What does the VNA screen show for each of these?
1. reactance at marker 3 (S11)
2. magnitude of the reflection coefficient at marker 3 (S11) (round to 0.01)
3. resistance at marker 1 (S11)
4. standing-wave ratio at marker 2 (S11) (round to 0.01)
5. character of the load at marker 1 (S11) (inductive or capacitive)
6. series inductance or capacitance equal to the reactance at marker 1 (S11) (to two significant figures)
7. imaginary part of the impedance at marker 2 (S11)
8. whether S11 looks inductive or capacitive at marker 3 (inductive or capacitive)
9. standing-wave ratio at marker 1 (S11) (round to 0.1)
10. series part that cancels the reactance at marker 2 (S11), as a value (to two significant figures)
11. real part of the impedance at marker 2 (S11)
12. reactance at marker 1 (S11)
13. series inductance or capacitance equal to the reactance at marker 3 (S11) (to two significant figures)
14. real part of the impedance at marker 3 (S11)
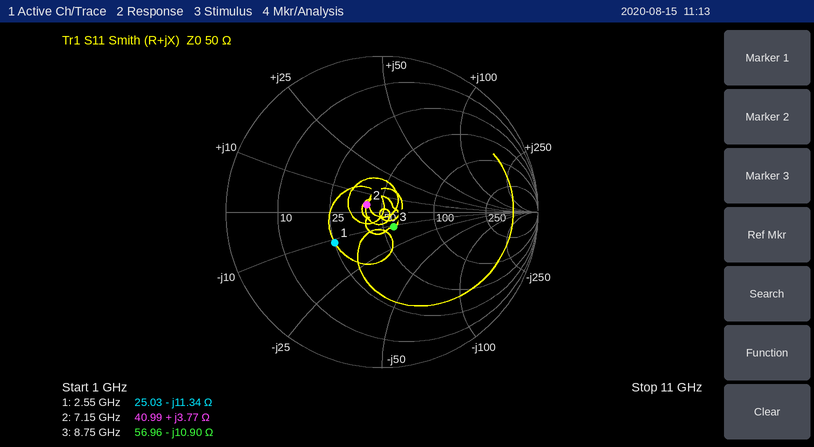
-10.90 Ω
0.12
25.03 Ω
1.24
capacitive
5.5 pF
+3.77 Ω
capacitive
2.1
5.9 pF
40.99 Ω
-11.34 Ω
1.7 pF
56.96 Ω
